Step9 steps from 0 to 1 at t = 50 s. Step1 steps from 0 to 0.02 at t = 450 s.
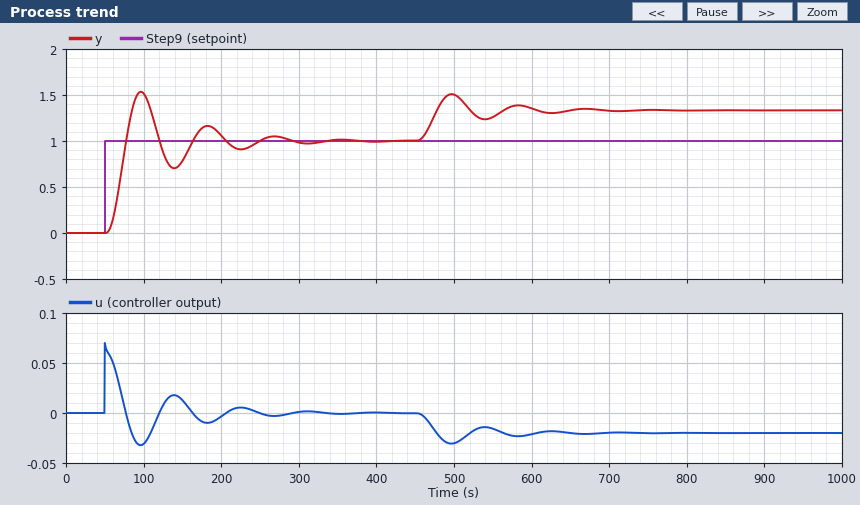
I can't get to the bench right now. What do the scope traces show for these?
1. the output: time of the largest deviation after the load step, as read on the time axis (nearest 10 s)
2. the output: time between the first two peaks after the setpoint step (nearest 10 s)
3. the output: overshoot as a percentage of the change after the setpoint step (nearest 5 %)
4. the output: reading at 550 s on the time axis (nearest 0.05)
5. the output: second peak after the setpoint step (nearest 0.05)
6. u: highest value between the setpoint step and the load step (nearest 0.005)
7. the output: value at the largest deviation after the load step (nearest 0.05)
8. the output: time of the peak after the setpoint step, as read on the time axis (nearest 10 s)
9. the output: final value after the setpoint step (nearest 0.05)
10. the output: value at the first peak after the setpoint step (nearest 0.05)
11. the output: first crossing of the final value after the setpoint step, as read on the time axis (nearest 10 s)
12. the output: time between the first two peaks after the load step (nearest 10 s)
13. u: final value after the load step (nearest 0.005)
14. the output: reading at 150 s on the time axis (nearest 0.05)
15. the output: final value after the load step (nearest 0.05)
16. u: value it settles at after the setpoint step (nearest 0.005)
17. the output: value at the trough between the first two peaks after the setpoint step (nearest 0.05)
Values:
500 s
90 s
55 %
1.25
1.15
0.070
1.50
100 s
1.00
1.55
80 s
90 s
-0.020
0.80
1.35
0.000
0.70
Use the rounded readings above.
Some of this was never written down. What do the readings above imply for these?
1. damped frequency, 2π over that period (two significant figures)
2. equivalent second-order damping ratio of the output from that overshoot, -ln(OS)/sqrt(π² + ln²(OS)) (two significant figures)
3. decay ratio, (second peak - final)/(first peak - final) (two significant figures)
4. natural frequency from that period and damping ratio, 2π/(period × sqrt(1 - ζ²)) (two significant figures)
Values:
0.070 rad/s
0.19
0.27
0.071 rad/s
